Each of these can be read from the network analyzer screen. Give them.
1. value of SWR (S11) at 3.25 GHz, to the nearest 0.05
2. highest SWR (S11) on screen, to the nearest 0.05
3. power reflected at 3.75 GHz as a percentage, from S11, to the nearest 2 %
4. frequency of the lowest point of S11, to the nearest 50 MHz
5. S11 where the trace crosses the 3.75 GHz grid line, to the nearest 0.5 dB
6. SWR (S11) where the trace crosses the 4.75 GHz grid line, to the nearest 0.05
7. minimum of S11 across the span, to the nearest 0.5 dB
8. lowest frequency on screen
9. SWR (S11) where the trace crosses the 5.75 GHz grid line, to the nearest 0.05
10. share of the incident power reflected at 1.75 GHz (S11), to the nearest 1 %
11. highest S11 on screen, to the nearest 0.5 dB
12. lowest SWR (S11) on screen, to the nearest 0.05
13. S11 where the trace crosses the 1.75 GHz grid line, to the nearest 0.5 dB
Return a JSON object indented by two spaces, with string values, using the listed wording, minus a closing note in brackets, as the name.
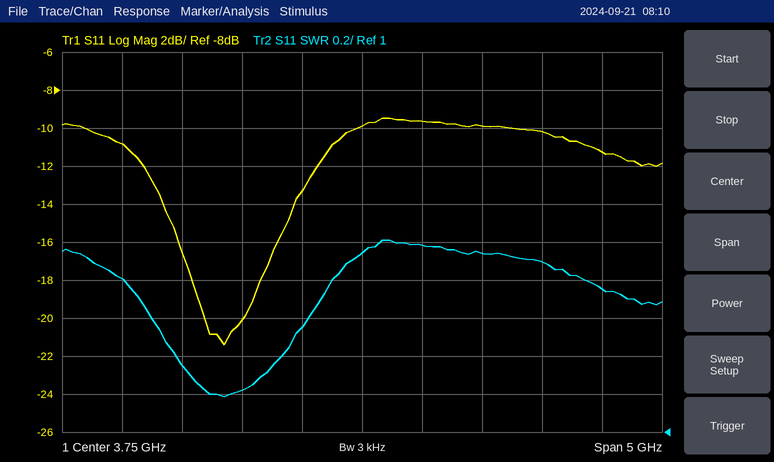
{
  "value of SWR (S11) at 3.25 GHz, to the nearest 0.05": "1.55",
  "highest SWR (S11) on screen, to the nearest 0.05": "2.00",
  "power reflected at 3.75 GHz as a percentage, from S11, to the nearest 2 %": "10 %",
  "frequency of the lowest point of S11, to the nearest 50 MHz": "2.60 GHz",
  "S11 where the trace crosses the 3.75 GHz grid line, to the nearest 0.5 dB": "-10.0 dB",
  "SWR (S11) where the trace crosses the 4.75 GHz grid line, to the nearest 0.05": "1.95",
  "minimum of S11 across the span, to the nearest 0.5 dB": "-21.5 dB",
  "lowest frequency on screen": "1.25 GHz",
  "SWR (S11) where the trace crosses the 5.75 GHz grid line, to the nearest 0.05": "1.75",
  "share of the incident power reflected at 1.75 GHz (S11), to the nearest 1 %": "8 %",
  "highest S11 on screen, to the nearest 0.5 dB": "-9.5 dB",
  "lowest SWR (S11) on screen, to the nearest 0.05": "1.20",
  "S11 where the trace crosses the 1.75 GHz grid line, to the nearest 0.5 dB": "-11.0 dB"
}
